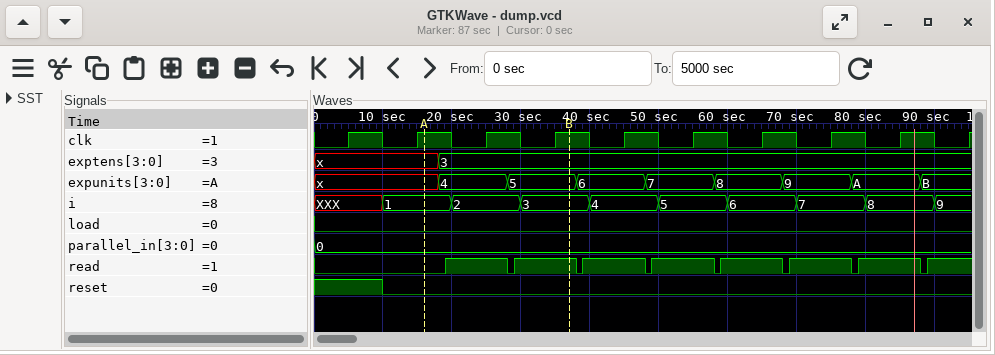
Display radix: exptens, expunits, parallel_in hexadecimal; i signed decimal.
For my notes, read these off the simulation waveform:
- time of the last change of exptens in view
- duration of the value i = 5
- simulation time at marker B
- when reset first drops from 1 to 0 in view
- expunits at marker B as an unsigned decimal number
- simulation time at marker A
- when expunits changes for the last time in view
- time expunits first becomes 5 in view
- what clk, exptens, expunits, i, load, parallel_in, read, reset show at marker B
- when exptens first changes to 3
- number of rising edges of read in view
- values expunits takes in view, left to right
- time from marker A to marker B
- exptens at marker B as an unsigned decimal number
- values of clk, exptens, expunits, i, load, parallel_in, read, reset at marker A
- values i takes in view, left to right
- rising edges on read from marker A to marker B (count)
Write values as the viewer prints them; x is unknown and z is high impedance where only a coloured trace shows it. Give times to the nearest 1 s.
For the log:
18 s
10 s
37 s
10 s
5
16 s
88 s
28 s
clk=1, exptens=3, expunits=5, i=3, load=0, parallel_in=0, read=1, reset=0
18 s
8
x, 4, 5, 6, 7, 8, 9, A, B
21 s
3
clk=1, exptens=x, expunits=x, i=1, load=0, parallel_in=0, read=0, reset=0
XXX, 1, 2, 3, 4, 5, 6, 7, 8, 9
2
